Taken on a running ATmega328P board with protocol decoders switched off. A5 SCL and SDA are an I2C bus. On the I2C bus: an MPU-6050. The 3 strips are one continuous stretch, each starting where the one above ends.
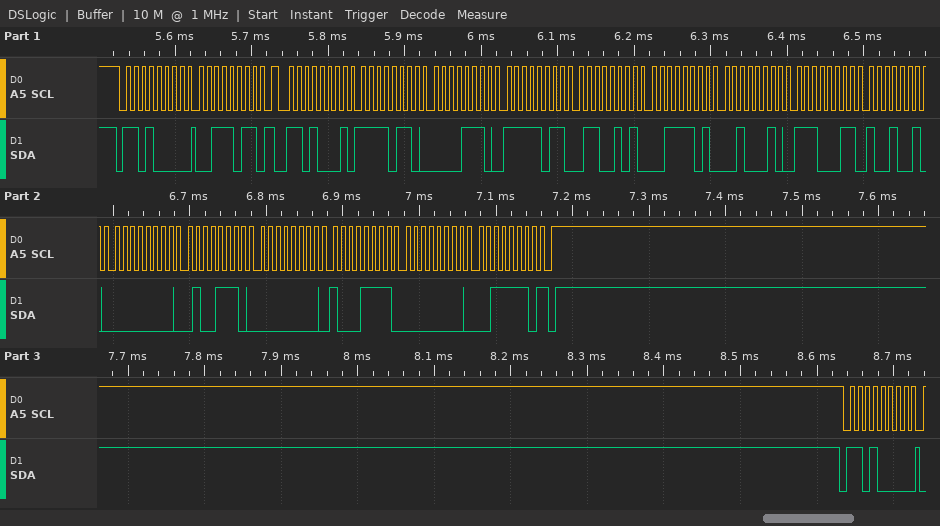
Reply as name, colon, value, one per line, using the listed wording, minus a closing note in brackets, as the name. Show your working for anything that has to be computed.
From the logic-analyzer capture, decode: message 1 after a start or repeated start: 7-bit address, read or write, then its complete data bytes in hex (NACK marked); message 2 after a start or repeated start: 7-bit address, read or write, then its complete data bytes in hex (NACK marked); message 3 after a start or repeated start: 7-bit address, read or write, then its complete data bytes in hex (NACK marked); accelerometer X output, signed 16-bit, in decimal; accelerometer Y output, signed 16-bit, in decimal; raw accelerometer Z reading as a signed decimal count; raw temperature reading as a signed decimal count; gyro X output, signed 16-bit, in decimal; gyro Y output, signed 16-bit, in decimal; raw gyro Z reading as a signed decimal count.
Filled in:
message 1 after a start or repeated start: 7-bit address, read or write, then its complete data bytes in hex: 0x68 write: 3B
message 2 after a start or repeated start: 7-bit address, read or write, then its complete data bytes in hex: 0x68 read: F6 0E FB 65 3D 22 E3 92 00 4E 00 8F 00 3E NACK
message 3 after a start or repeated start: 7-bit address, read or write, then its complete data bytes in hex: 0x68 write
accelerometer X output, signed 16-bit, in decimal: 0xF60E = -2546
accelerometer Y output, signed 16-bit, in decimal: 0xFB65 = -1179
raw accelerometer Z reading as a signed decimal count: 0x3D22 = 15650
raw temperature reading as a signed decimal count: 0xE392 = -7278
gyro X output, signed 16-bit, in decimal: 0x004E = 78
gyro Y output, signed 16-bit, in decimal: 0x008F = 143
raw gyro Z reading as a signed decimal count: 0x003E = 62
